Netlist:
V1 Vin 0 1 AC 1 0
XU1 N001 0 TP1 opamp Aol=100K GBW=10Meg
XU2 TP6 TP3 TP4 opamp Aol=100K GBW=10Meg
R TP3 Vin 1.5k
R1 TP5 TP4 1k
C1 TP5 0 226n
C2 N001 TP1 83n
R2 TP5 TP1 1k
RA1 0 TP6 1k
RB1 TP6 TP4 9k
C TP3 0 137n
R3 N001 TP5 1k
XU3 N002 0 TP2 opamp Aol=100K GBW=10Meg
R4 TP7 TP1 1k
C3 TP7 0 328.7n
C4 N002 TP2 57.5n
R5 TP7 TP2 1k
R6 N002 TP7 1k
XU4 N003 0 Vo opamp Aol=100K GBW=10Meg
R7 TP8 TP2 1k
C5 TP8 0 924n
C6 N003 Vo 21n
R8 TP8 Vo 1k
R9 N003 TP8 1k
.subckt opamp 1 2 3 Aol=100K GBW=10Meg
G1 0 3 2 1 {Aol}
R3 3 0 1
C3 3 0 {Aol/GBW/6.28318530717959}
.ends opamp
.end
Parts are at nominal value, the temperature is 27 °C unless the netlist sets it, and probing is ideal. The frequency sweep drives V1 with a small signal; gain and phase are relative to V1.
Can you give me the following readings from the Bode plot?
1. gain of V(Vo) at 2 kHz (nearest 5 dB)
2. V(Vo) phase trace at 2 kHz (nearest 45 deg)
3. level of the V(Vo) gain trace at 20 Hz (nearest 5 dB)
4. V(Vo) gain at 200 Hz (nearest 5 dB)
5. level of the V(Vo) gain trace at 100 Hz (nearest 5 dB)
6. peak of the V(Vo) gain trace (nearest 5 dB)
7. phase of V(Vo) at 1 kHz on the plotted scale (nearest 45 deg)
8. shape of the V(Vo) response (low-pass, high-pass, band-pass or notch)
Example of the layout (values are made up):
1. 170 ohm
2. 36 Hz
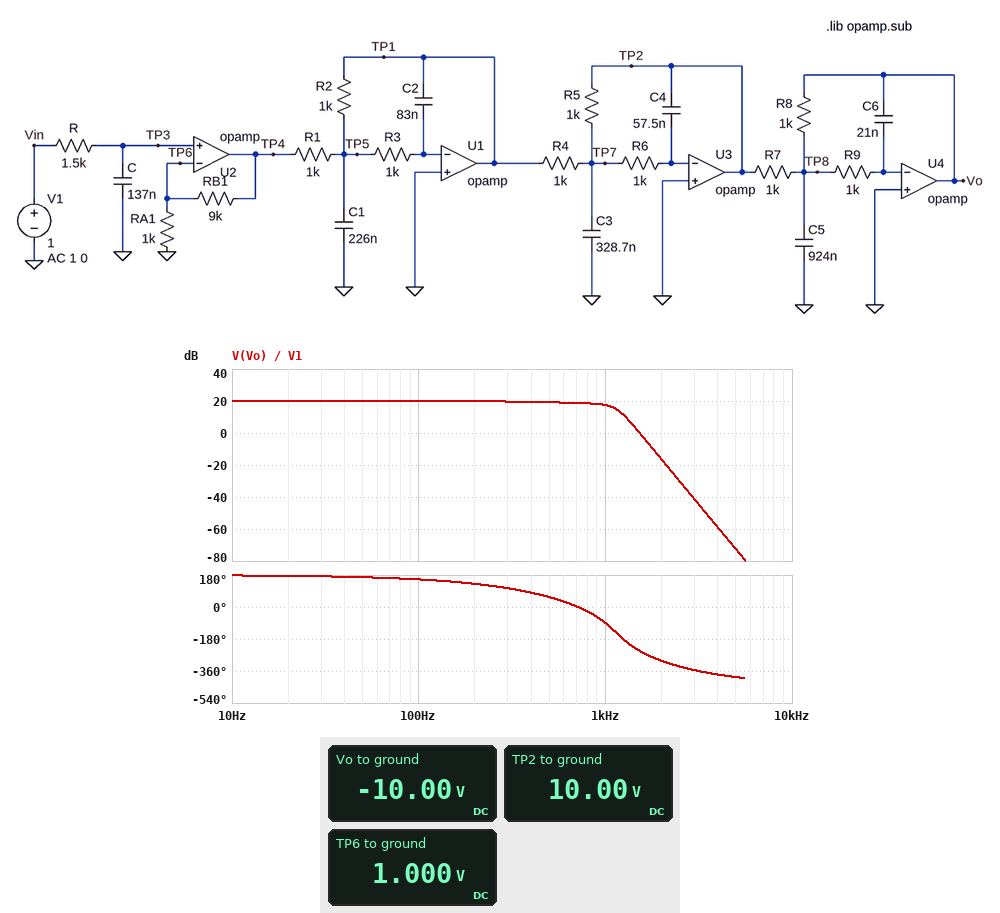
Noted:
1. -15 dB
2. -315 deg
3. 20 dB
4. 20 dB
5. 20 dB
6. 20 dB
7. -90 deg
8. low-pass
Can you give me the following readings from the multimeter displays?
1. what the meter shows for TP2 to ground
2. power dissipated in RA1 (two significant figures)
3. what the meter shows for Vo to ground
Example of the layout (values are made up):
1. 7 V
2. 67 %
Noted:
1. 10.00 V
2. 1.0 mW
3. -10.00 V
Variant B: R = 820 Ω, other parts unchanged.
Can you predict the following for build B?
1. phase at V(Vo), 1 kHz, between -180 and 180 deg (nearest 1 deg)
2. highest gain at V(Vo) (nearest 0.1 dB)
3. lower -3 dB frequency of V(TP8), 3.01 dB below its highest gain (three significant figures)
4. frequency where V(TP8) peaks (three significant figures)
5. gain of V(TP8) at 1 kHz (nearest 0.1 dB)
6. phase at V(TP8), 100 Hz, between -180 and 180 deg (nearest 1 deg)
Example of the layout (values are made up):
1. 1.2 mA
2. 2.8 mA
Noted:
1. -72 deg
2. 20.5 dB
3. 682 Hz
4. 1.01 kHz
5. 2.5 dB
6. 68 deg
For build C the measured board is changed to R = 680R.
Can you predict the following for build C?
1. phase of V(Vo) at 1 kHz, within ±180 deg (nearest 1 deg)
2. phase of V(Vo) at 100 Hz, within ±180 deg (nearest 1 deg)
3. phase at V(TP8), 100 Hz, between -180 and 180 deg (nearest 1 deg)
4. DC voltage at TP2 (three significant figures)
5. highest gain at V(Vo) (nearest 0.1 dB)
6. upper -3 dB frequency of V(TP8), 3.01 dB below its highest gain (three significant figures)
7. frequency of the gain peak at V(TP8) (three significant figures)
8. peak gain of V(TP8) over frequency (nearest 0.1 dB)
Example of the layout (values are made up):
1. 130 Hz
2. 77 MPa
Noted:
1. -67 deg
2. 159 deg
3. 69 deg
4. 10.0 V
5. 20.9 dB
6. 1.23 kHz
7. 1.02 kHz
8. 3.0 dB
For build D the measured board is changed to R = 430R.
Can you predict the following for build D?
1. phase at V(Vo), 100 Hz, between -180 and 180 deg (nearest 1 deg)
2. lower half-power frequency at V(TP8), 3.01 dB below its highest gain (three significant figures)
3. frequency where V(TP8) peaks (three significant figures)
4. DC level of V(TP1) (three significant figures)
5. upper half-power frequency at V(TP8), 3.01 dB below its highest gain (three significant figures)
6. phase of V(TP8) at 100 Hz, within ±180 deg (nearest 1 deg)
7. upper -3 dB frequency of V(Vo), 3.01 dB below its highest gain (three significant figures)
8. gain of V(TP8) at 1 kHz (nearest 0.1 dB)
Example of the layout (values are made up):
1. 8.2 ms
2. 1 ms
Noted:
1. 160 deg
2. 722 Hz
3. 1.03 kHz
4. -10.0 V
5. 1.24 kHz
6. 70 deg
7. 1.17 kHz
8. 3.7 dB
